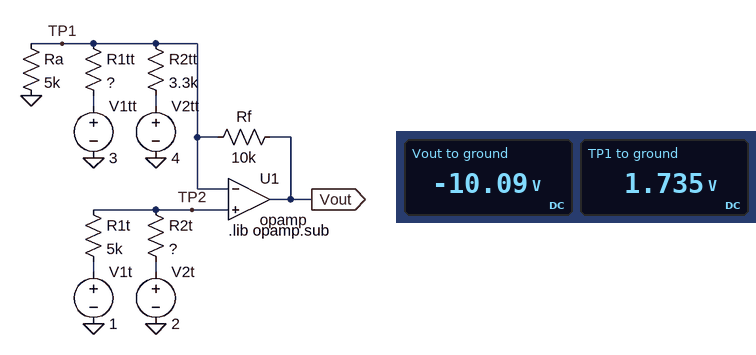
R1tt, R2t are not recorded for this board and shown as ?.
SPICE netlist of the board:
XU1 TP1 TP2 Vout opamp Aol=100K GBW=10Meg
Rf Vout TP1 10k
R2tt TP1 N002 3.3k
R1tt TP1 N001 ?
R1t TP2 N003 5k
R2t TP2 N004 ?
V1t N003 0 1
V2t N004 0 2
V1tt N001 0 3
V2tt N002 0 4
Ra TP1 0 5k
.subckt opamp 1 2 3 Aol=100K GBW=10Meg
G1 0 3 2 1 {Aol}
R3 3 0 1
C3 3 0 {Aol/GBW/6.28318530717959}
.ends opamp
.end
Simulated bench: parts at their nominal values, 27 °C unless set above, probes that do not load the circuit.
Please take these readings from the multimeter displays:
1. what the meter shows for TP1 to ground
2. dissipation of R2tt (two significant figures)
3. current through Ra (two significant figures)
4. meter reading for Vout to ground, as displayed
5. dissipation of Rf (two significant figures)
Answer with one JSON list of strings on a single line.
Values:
["1.735 V", "1.6 mW", "350 µA", "-10.09 V", "14 mW"]
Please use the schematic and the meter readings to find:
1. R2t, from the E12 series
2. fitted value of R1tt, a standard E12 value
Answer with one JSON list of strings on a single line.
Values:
["1.8 kΩ", "1.5 kΩ"]
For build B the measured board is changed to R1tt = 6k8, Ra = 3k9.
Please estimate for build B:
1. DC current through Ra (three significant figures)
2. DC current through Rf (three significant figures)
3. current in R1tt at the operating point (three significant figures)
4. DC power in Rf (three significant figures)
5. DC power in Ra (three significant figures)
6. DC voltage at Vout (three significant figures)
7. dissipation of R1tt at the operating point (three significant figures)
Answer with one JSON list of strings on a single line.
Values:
["445 µA", "427 µA", "186 µA", "1.83 mW", "772 µW", "-2.54 V", "235 µW"]
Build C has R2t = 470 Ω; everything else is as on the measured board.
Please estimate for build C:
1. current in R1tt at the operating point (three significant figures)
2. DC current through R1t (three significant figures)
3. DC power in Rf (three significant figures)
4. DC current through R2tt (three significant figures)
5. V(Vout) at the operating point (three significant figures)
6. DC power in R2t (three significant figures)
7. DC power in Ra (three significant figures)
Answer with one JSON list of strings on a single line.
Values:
["724 µA", "183 µA", "9.47 mW", "632 µA", "-7.82 V", "15.7 µW", "733 µW"]
